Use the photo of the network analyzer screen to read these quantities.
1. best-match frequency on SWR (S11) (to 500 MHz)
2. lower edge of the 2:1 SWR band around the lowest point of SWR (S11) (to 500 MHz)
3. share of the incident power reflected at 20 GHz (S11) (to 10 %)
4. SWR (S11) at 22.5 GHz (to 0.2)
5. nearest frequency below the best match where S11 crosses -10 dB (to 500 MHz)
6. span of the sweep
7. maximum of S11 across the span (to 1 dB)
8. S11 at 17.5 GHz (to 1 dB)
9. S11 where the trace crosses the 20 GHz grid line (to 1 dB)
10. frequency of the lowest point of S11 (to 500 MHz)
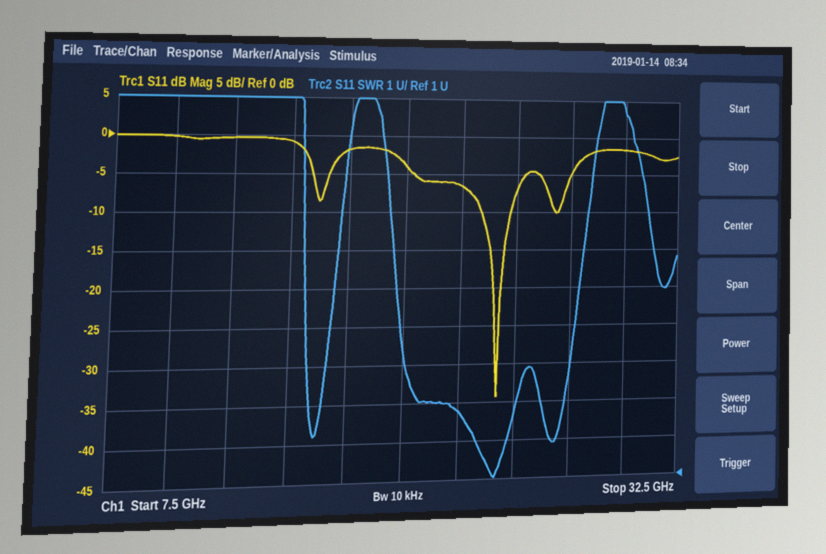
24.0 GHz
23.5 GHz
40 %
2.8
23.5 GHz
25 GHz
0 dB
-2 dB
-4 dB
24.0 GHz
